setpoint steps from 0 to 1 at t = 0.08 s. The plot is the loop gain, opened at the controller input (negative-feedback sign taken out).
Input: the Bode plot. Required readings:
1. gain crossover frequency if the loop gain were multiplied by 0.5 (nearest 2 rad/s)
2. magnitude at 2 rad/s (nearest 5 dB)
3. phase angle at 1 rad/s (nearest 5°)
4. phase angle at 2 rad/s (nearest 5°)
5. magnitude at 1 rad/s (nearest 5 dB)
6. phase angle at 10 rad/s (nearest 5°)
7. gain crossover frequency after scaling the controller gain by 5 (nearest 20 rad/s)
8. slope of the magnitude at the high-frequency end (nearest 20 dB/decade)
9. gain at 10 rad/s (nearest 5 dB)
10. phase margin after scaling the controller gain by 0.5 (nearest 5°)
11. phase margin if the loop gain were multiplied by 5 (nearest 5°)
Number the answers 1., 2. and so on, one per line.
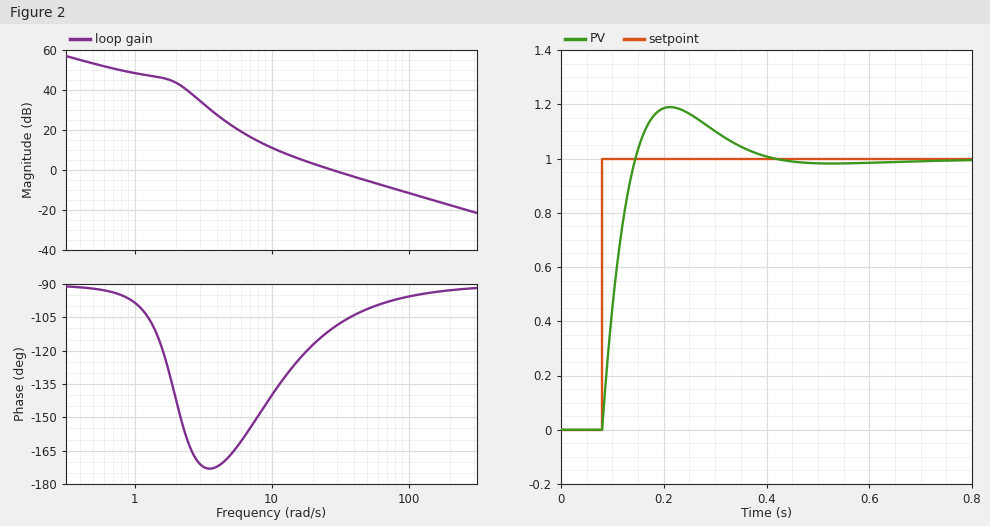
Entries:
1. 16 rad/s
2. 45 dB
3. -100°
4. -140°
5. 50 dB
6. -140°
7. 140 rad/s
8. -20 dB/decade
9. 10 dB
10. 55°
11. 85°
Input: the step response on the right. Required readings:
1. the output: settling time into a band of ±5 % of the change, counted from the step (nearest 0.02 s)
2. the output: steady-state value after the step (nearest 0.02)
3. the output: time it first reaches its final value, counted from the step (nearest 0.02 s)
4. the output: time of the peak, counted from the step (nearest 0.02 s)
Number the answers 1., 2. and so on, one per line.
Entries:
1. 0.26 s
2. 1.00
3. 0.06 s
4. 0.14 s
